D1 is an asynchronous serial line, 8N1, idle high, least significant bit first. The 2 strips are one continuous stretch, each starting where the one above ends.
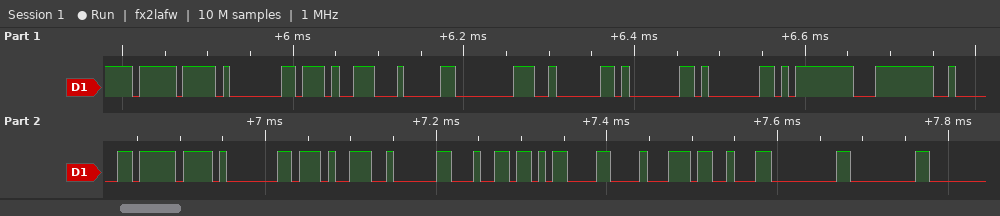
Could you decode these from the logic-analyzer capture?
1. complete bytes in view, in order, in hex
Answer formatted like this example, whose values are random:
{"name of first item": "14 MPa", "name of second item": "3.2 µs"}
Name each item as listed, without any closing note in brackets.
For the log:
{"complete bytes in view, in order, in hex": "0xDF 0x01 0x97 0x04 0x80 0x02 0x01 0x01 0xFD 0xFC 0x02 0xDF 0x01 0x97 0x02 0x64 0x0D 0x88 0x13 0x00 0x00"}
